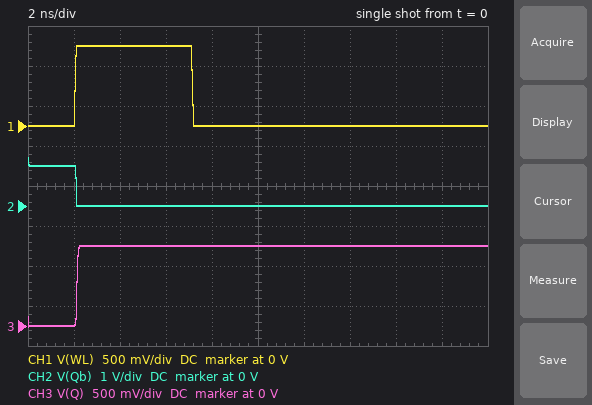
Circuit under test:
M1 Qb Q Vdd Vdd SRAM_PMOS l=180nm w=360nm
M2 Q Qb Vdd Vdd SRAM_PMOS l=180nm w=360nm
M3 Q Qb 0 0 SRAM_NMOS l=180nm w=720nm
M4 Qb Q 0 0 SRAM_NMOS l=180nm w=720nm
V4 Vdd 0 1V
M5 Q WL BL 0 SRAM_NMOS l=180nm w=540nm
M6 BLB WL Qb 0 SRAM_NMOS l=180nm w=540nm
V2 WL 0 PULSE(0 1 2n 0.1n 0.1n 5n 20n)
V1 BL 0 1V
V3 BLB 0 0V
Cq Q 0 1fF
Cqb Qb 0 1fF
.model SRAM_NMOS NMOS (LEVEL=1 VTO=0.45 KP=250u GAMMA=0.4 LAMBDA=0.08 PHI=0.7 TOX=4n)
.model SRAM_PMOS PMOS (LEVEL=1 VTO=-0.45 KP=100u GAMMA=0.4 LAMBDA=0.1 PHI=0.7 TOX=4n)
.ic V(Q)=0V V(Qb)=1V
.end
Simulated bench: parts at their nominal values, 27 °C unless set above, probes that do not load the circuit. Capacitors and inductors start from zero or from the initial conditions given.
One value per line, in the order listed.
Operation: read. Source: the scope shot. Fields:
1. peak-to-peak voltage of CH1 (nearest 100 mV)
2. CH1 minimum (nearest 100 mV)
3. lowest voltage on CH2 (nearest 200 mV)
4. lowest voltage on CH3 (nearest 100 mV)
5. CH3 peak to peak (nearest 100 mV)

1.0 V
0 V
0 V
0 V
1.0 V
